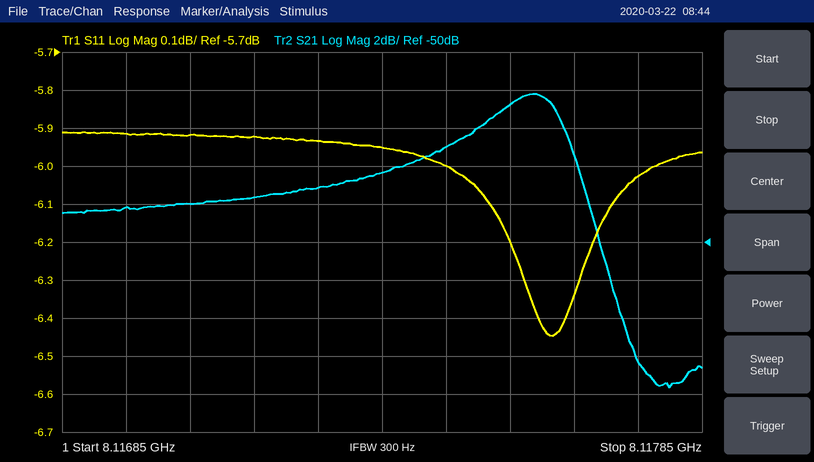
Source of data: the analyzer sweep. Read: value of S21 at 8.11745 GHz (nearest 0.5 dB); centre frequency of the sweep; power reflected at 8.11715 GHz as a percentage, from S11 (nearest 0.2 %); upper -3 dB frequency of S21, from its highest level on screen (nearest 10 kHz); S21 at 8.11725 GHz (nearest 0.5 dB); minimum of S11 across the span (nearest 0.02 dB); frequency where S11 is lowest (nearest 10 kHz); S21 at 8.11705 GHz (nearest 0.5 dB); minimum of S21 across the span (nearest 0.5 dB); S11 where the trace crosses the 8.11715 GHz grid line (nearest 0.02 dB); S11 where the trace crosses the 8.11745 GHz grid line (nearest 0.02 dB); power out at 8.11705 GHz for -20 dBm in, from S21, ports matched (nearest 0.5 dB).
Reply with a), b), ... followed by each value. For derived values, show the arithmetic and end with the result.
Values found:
a) -45.0 dB
b) 8.11735 GHz
c) 10^(-5.92/10) ≈ 25.6 %
d) 8.11765 GHz
e) -47.0 dB
f) -6.44 dB
g) 8.11762 GHz
h) -48.0 dB
i) -57.5 dB
j) -5.92 dB
k) -6.00 dB
l) -20 dBm + (-48.0 dB) = -68.0 dBm
